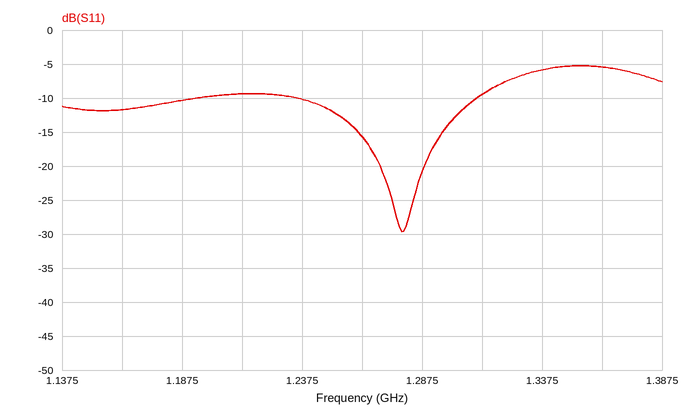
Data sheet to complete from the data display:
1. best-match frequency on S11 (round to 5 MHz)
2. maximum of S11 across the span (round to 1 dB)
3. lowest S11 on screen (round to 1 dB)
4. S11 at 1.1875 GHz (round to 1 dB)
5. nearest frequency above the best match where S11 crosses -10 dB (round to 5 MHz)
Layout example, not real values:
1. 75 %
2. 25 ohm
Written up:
1. 1.280 GHz
2. -5 dB
3. -30 dB
4. -10 dB
5. 1.310 GHz
